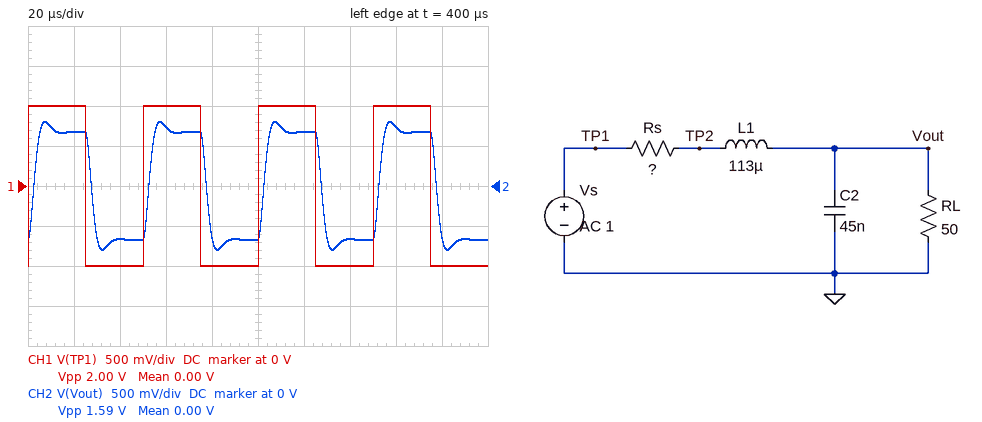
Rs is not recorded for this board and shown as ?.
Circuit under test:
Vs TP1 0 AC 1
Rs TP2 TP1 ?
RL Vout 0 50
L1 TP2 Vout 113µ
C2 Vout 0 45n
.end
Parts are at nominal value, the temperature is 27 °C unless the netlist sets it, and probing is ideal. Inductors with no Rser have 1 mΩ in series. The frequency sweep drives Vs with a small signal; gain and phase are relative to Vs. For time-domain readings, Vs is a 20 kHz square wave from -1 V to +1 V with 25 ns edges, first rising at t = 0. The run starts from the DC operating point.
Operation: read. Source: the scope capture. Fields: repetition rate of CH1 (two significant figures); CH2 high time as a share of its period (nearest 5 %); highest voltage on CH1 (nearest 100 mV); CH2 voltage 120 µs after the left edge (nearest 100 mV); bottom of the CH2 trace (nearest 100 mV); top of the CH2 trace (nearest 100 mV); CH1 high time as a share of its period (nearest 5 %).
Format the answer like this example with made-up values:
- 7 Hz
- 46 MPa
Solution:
- 20 kHz
- 50 %
- 1.0 V
- 700 mV
- -800 mV
- 800 mV
- 50 %
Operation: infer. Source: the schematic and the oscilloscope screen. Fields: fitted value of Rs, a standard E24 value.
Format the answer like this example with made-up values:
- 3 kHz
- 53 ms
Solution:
- 24 Ω
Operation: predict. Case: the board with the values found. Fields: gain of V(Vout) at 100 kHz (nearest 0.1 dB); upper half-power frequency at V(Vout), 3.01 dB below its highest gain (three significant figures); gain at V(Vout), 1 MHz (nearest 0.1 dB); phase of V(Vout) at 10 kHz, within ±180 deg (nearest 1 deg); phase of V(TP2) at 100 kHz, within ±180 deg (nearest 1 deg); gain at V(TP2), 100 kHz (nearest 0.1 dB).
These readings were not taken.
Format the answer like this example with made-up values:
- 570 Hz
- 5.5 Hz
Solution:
- -6.7 dB
- 95.0 kHz
- -46.0 dB
- -8 deg
- 21 deg
- -1.9 dB
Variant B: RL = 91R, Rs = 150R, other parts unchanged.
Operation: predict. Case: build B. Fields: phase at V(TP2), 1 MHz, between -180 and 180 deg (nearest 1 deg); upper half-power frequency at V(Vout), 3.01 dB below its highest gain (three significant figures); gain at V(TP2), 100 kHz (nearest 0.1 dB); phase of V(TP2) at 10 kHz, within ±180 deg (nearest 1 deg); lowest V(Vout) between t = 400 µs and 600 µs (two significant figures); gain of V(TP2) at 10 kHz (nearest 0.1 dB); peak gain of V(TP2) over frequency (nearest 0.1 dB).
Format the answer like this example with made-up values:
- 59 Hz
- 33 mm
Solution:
- 12 deg
- 65.6 kHz
- -12.0 dB
- -6 deg
- -380 mV
- -8.7 dB
- 0 dB
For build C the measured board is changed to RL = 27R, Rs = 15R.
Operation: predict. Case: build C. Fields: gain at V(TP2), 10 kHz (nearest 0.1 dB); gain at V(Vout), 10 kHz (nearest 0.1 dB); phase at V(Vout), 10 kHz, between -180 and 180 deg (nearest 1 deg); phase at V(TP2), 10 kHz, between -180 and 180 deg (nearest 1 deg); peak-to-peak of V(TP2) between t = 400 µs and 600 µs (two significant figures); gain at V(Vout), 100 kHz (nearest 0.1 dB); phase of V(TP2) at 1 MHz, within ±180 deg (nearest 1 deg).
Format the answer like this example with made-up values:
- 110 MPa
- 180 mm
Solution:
- -3.8 dB
- -3.9 dB
- -11 deg
- 4 deg
- 2.7 V
- -9.8 dB
- 1 deg
